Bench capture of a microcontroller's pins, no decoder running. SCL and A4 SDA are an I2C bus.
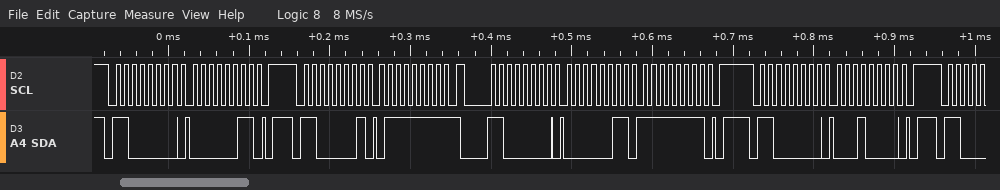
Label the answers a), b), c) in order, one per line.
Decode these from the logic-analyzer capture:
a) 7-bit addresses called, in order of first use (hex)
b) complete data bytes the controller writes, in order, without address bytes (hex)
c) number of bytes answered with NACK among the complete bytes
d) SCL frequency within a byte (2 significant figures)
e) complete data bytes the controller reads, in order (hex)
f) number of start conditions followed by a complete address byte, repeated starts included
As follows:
a) 0x60
b) 03 03 FF 10
c) 1
d) 100 kHz
e) 7F
f) 4
